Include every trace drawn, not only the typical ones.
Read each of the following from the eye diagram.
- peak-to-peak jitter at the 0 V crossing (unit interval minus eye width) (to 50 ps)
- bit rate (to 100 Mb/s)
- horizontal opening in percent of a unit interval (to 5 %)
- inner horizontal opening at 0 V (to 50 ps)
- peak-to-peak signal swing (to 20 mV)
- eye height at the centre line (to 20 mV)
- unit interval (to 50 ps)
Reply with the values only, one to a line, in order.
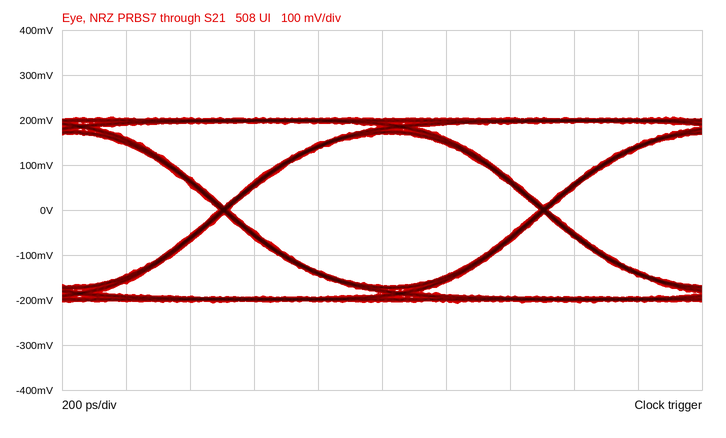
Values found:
50 ps
1.0 Gb/s
95 %
950 ps
420 mV
340 mV
1.00 ns
